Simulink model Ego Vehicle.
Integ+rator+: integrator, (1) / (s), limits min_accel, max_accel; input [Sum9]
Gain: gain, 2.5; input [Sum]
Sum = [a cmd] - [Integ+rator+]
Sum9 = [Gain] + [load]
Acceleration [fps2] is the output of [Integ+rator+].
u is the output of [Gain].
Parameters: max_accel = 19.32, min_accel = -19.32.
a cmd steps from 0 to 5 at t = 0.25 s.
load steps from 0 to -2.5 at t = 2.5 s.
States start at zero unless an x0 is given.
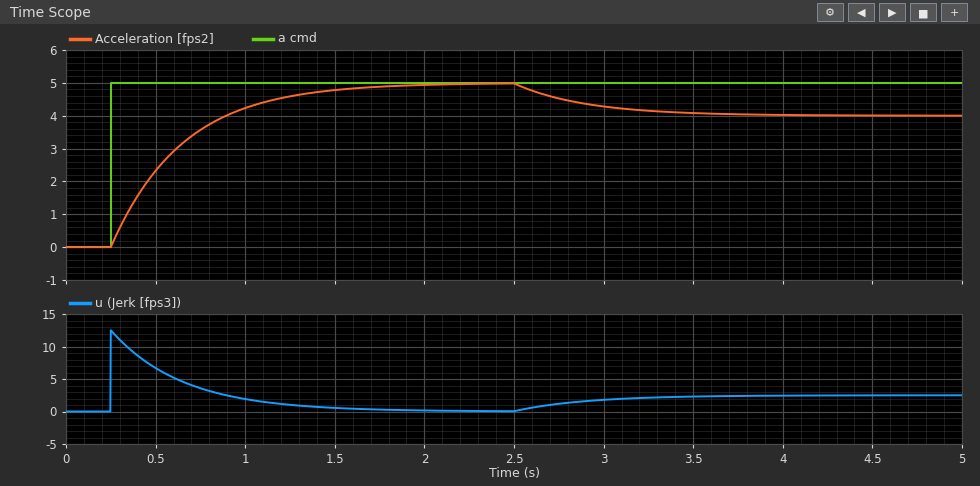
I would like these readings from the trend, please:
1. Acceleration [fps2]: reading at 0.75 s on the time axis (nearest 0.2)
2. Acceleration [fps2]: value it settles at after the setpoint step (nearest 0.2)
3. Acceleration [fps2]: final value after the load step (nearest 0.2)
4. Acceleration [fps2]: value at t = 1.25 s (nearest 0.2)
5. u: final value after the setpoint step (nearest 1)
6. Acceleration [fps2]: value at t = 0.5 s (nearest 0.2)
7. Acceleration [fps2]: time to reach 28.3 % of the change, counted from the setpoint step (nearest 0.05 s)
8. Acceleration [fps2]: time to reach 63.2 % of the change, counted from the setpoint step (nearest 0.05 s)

3.6
5.0
4.0
4.6
0
2.4
0.15 s
0.40 s
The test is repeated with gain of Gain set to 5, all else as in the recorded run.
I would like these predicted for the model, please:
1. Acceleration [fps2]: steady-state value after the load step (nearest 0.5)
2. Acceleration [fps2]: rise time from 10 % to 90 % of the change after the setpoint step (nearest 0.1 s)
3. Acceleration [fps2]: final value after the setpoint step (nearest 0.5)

4.5
0.4 s
5.0
